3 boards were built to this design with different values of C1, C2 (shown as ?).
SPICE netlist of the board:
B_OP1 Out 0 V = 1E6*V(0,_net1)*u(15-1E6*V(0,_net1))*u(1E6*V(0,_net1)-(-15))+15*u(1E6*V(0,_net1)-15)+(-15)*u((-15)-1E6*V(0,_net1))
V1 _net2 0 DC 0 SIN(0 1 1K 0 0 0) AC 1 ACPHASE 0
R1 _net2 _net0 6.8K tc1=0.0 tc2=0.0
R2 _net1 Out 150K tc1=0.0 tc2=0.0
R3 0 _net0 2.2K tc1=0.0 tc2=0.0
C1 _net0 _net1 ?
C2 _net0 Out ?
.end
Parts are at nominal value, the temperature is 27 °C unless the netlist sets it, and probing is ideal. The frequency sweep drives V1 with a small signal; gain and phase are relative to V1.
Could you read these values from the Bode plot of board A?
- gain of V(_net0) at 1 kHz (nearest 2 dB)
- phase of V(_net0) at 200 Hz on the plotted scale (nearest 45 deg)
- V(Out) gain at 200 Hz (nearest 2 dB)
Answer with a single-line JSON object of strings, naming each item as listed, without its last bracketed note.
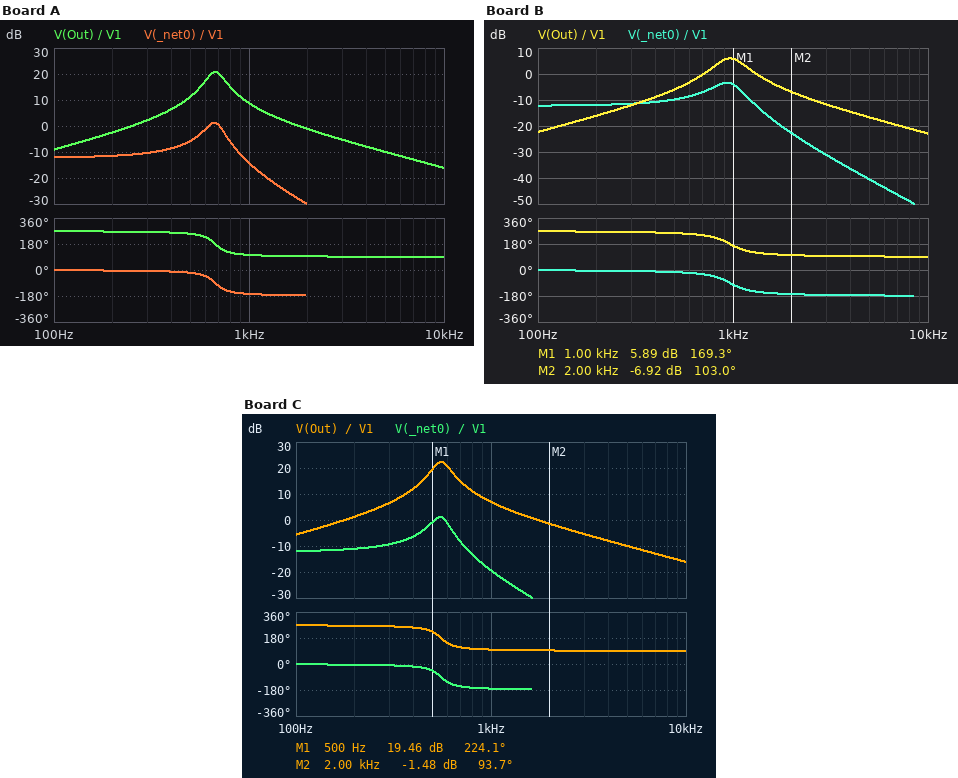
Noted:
{"gain of V(_net0) at 1 kHz": "-14 dB", "phase of V(_net0) at 200 Hz on the plotted scale": "0 deg", "V(Out) gain at 200 Hz": "-2 dB"}
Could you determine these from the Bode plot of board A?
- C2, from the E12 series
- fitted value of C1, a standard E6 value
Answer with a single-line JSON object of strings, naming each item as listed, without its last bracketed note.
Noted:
{"C2, from the E12 series": "15 nF", "fitted value of C1, a standard E6 value": "15 nF"}
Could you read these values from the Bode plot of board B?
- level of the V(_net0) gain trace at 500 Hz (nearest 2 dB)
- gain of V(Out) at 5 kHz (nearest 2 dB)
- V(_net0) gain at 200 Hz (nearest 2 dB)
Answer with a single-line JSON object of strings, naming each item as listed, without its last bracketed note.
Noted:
{"level of the V(_net0) gain trace at 500 Hz": "-10 dB", "gain of V(Out) at 5 kHz": "-16 dB", "V(_net0) gain at 200 Hz": "-12 dB"}
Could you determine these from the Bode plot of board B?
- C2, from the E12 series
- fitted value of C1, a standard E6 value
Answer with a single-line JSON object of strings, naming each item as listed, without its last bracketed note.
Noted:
{"C2, from the E12 series": "33 nF", "fitted value of C1, a standard E6 value": "3.3 nF"}
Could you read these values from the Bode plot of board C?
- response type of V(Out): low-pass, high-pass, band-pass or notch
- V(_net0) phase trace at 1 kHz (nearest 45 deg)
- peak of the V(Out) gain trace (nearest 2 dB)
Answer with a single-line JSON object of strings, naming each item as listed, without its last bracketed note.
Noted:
{"response type of V(Out): low-pass, high-pass, band-pass or notch": "band-pass", "V(_net0) phase trace at 1 kHz": "-180 deg", "peak of the V(Out) gain trace": "22 dB"}
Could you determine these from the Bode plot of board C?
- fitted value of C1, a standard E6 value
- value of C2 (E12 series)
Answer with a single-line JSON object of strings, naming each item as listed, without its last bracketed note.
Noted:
{"fitted value of C1, a standard E6 value": "22 nF", "value of C2": "15 nF"}
